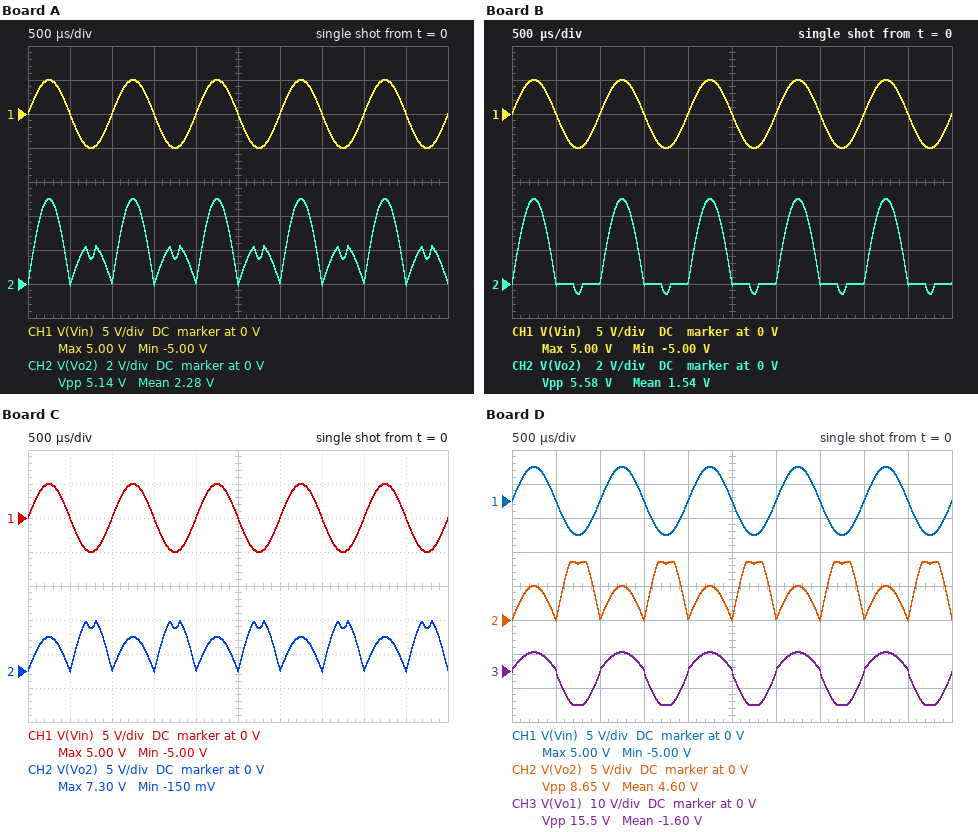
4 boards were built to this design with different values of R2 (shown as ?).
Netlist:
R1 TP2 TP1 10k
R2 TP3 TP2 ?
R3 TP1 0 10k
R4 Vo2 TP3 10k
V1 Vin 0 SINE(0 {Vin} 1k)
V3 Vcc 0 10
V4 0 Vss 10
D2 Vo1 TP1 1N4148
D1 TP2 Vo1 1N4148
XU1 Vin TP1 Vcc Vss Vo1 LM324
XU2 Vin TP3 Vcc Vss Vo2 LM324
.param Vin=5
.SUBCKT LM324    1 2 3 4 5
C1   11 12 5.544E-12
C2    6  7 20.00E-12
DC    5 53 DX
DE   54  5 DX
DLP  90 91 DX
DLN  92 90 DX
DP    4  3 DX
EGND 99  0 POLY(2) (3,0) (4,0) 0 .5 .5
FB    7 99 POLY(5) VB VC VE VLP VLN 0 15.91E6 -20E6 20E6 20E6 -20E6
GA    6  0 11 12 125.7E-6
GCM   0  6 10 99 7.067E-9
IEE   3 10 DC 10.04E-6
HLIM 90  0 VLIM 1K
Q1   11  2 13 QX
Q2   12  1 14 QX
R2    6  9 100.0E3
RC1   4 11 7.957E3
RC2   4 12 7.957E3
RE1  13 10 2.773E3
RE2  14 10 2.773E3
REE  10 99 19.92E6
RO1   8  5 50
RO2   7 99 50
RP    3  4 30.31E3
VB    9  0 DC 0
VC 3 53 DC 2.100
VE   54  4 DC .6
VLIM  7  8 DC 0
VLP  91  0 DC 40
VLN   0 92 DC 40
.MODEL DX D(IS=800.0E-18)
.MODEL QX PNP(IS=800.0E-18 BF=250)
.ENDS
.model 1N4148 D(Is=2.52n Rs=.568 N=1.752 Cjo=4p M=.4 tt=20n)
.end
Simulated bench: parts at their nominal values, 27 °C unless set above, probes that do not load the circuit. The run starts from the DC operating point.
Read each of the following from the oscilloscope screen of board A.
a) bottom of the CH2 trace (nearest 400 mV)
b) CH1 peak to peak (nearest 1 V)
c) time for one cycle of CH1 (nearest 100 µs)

0 V
10 V
1.0 ms
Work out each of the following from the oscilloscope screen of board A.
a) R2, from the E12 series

6.8 kΩ
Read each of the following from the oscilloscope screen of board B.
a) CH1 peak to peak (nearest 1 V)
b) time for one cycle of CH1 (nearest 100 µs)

10 V
1.0 ms
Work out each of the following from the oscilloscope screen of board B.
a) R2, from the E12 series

10 kΩ
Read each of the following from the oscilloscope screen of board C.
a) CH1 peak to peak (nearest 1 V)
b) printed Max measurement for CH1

10 V
5.00 V
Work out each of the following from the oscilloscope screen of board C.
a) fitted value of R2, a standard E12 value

3.9 kΩ
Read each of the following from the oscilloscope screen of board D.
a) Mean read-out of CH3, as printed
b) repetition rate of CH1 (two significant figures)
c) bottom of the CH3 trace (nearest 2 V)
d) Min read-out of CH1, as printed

-1.60 V
1.0 kHz
-10 V
-5.00 V
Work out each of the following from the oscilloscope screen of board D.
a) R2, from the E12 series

3.3 kΩ
